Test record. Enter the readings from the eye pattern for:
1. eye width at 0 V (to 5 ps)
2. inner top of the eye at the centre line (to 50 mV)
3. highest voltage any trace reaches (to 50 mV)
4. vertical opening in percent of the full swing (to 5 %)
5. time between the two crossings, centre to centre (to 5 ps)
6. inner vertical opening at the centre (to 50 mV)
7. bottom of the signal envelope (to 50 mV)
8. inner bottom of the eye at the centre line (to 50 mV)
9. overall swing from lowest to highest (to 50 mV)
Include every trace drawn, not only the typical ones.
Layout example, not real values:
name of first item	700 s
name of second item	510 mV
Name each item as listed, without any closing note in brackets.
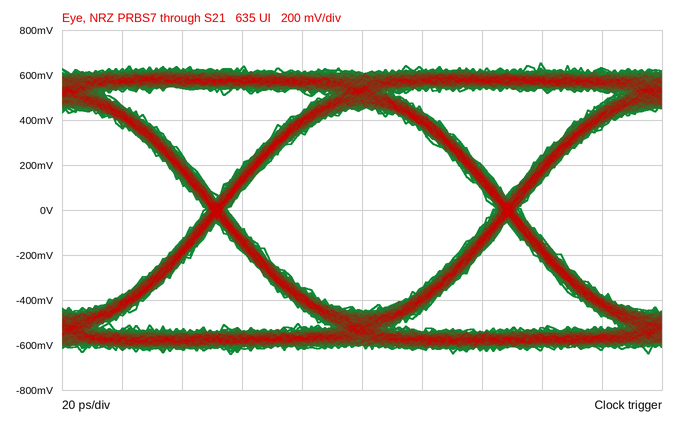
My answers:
eye width at 0 V	90 ps
inner top of the eye at the centre line	450 mV
highest voltage any trace reaches	650 mV
vertical opening in percent of the full swing	70 %
time between the two crossings, centre to centre	95 ps
inner vertical opening at the centre	900 mV
bottom of the signal envelope	-650 mV
inner bottom of the eye at the centre line	-450 mV
overall swing from lowest to highest	1.30 V
